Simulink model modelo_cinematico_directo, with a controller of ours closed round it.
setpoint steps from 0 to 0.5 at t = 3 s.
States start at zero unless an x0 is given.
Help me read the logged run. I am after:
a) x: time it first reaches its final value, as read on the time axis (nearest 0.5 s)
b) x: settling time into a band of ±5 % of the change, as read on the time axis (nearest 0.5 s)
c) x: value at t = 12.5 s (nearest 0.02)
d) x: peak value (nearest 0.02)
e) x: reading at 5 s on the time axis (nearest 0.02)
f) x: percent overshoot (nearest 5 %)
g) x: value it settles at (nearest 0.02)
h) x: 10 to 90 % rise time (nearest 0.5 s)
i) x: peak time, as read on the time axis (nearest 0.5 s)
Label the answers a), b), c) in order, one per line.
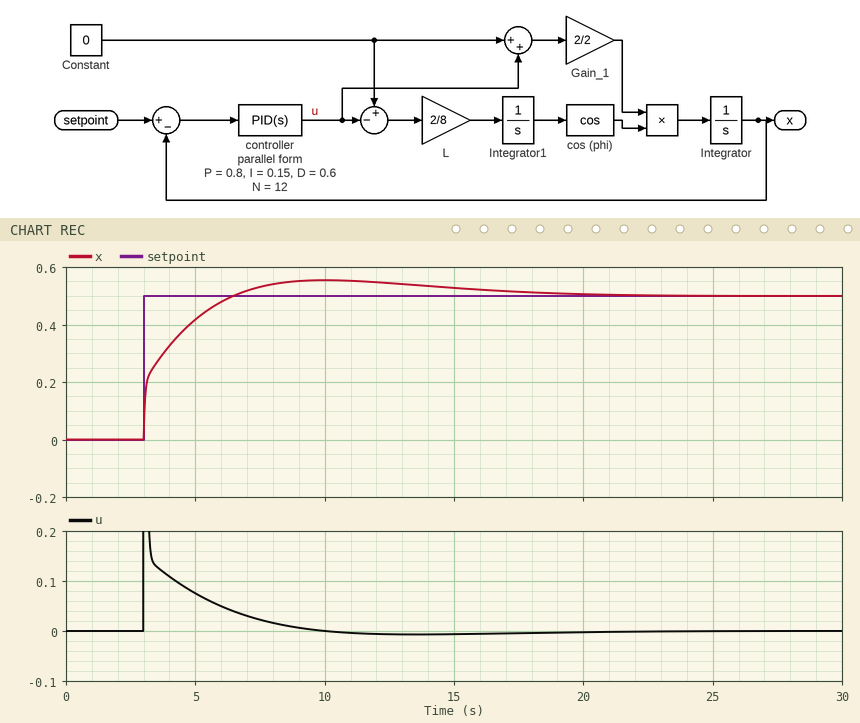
a) 6.5 s
b) 15.5 s
c) 0.54
d) 0.56
e) 0.42
f) 10 %
g) 0.50
h) 2.5 s
i) 10.0 s
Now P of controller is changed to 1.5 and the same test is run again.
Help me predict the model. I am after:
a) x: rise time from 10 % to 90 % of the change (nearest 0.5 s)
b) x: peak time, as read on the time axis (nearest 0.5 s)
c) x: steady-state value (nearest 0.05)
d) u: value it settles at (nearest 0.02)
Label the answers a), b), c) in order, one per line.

a) 1.5 s
b) 8.5 s
c) 0.50
d) 0.00
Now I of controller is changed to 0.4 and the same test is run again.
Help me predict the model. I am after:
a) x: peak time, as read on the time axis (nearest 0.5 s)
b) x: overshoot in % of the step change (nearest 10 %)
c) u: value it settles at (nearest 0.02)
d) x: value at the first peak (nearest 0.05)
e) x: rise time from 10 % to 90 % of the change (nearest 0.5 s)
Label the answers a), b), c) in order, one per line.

a) 8.0 s
b) 20 %
c) 0.00
d) 0.60
e) 2.0 s
